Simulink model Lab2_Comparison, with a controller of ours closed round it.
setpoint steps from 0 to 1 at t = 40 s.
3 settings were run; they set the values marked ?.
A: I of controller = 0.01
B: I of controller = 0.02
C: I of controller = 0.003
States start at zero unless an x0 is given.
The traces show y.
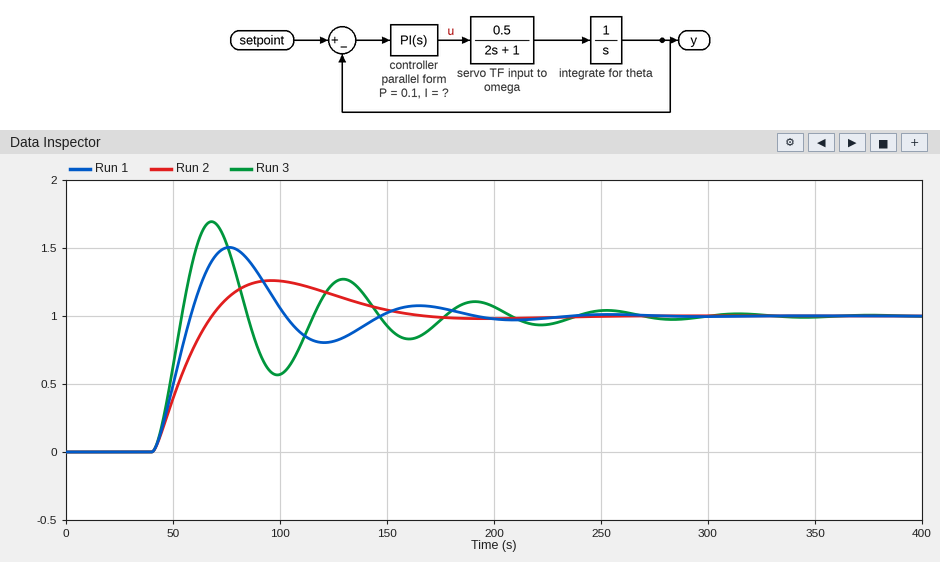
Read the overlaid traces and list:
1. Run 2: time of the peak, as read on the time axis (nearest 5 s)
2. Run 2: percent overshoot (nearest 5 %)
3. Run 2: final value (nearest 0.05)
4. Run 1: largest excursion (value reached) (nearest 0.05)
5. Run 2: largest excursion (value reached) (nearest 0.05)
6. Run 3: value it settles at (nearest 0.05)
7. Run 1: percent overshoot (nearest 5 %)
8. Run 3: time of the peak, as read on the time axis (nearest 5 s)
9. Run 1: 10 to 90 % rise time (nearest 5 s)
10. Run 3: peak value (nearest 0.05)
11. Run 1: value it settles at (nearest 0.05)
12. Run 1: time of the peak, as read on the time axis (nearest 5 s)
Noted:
95 s
25 %
1.00
1.50
1.25
1.00
50 %
70 s
15 s
1.70
1.00
75 s
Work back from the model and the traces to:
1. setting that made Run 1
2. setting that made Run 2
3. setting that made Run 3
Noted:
A
C
B
